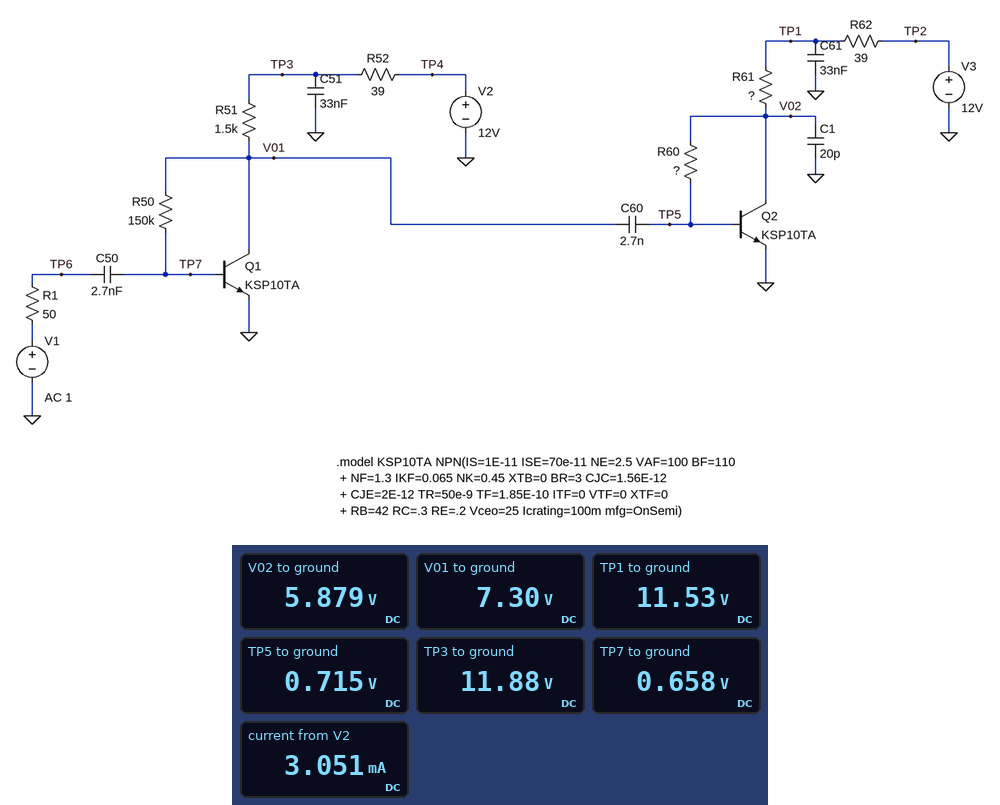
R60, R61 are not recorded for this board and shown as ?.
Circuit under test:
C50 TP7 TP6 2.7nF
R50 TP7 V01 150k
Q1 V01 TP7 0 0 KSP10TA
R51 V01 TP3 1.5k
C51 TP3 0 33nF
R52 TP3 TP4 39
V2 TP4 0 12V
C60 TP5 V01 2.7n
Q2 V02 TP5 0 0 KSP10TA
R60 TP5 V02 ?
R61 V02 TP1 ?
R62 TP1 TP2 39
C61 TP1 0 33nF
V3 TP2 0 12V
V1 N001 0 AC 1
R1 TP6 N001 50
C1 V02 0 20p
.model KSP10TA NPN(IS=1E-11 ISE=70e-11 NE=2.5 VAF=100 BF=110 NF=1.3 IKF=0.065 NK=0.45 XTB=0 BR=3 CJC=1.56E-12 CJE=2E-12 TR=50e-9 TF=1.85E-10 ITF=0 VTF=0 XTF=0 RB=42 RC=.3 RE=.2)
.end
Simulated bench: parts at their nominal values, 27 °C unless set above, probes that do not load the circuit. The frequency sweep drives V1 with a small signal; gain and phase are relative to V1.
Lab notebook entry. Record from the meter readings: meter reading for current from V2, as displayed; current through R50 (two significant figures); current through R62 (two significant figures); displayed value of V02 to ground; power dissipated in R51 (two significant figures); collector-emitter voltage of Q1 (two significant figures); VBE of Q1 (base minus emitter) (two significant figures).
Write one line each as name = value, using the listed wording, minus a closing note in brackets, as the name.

meter reading for current from V2, as displayed = 3.051 mA
current through R50 = 44 µA
current through R62 = 12 mA
displayed value of V02 to ground = 5.879 V
power dissipated in R51 = 14 mW
collector-emitter voltage of Q1 = 7.3 V
VBE of Q1 (base minus emitter) = 660 mV
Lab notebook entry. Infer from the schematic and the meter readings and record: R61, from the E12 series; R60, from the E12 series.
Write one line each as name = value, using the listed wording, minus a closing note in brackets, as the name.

R61, from the E12 series = 470 Ω
R60, from the E12 series = 33 kΩ
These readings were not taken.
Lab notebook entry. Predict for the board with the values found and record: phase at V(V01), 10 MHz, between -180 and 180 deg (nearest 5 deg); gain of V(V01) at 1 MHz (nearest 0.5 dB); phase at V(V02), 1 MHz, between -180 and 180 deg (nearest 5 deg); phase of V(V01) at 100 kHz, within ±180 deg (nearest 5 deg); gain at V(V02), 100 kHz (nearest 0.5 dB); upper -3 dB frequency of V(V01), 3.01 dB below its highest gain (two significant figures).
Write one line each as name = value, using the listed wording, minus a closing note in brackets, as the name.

phase at V(V01), 10 MHz, between -180 and 180 deg = 150 deg
gain of V(V01) at 1 MHz = 21.0 dB
phase at V(V02), 1 MHz, between -180 and 180 deg = -5 deg
phase of V(V01) at 100 kHz, within ±180 deg = 160 deg
gain at V(V02), 100 kHz = 60.0 dB
upper -3 dB frequency of V(V01), 3.01 dB below its highest gain = 130 kHz
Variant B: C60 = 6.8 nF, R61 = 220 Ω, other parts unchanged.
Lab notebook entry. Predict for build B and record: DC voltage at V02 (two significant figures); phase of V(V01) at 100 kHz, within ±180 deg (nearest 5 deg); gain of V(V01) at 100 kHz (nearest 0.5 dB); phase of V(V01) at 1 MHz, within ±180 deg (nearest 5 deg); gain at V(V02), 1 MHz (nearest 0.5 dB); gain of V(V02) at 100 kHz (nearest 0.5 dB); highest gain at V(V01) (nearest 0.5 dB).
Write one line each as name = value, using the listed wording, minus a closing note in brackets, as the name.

DC voltage at V02 = 7.7 V
phase of V(V01) at 100 kHz, within ±180 deg = 165 deg
gain of V(V01) at 100 kHz = 24.5 dB
phase of V(V01) at 1 MHz, within ±180 deg = 170 deg
gain at V(V02), 1 MHz = 57.0 dB
gain of V(V02) at 100 kHz = 56.5 dB
highest gain at V(V01) = 27.0 dB
